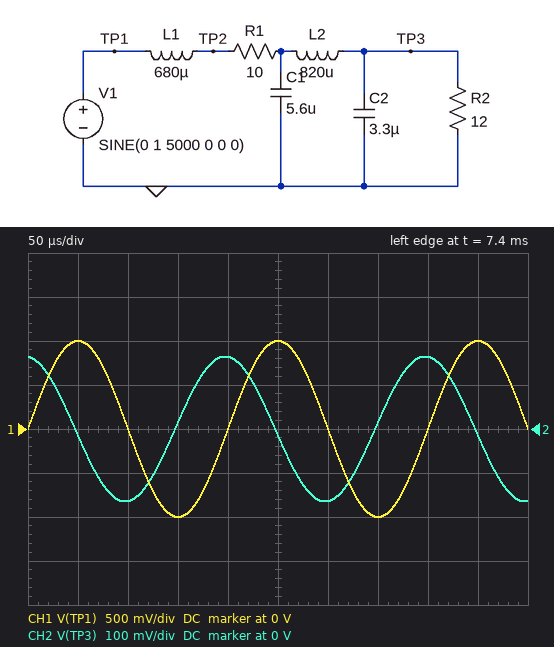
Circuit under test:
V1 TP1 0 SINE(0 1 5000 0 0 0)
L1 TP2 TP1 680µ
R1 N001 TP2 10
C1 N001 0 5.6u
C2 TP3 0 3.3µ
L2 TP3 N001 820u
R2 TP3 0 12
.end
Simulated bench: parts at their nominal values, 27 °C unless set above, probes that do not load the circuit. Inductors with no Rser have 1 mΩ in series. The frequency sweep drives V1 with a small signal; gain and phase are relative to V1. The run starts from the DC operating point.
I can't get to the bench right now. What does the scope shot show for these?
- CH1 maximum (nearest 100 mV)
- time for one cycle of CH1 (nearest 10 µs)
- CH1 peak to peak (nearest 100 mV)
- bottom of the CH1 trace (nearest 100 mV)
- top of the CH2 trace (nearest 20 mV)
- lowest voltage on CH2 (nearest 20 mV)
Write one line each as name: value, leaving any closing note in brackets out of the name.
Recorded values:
CH1 maximum: 1.0 V
time for one cycle of CH1: 200 µs
CH1 peak to peak: 2.0 V
bottom of the CH1 trace: -1.0 V
top of the CH2 trace: 160 mV
lowest voltage on CH2: -160 mV
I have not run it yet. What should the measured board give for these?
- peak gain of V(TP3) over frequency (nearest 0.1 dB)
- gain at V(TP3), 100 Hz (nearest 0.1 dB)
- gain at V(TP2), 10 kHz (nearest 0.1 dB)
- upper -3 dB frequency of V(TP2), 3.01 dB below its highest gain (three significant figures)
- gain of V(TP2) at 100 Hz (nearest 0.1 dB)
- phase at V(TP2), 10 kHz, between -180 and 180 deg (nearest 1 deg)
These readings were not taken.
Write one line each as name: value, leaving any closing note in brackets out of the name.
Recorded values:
peak gain of V(TP3) over frequency: -5.3 dB
gain at V(TP3), 100 Hz: -5.3 dB
gain at V(TP2), 10 kHz: -11.9 dB
upper -3 dB frequency of V(TP2), 3.01 dB below its highest gain: 4.70 kHz
gain of V(TP2) at 100 Hz: 0 dB
phase at V(TP2), 10 kHz, between -180 and 180 deg: -93 deg
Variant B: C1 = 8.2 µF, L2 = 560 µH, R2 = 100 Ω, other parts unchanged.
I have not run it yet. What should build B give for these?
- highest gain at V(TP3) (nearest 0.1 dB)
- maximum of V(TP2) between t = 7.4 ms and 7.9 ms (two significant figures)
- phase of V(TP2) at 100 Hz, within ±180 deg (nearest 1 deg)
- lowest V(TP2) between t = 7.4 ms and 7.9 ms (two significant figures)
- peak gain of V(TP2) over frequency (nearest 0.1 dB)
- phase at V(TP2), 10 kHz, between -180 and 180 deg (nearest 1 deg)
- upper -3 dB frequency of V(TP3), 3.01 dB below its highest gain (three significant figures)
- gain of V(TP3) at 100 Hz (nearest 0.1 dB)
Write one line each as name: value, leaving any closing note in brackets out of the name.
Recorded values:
highest gain at V(TP3): 3.5 dB
maximum of V(TP2) between t = 7.4 ms and 7.9 ms: 740 mV
phase of V(TP2) at 100 Hz, within ±180 deg: 0 deg
lowest V(TP2) between t = 7.4 ms and 7.9 ms: -740 mV
peak gain of V(TP2) over frequency: 1.9 dB
phase at V(TP2), 10 kHz, between -180 and 180 deg: -88 deg
upper -3 dB frequency of V(TP3), 3.01 dB below its highest gain: 4.70 kHz
gain of V(TP3) at 100 Hz: -0.8 dB
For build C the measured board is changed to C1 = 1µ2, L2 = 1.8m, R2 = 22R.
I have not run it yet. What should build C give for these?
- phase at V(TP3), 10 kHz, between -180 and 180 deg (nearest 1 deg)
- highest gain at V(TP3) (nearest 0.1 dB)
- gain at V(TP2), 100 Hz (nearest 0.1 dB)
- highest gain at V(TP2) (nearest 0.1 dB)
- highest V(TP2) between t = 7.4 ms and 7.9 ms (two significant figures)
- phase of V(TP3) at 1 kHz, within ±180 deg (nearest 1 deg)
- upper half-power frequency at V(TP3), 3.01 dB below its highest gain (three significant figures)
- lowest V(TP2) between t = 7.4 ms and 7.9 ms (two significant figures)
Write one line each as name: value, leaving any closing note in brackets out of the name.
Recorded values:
phase at V(TP3), 10 kHz, between -180 and 180 deg: 33 deg
highest gain at V(TP3): -3.1 dB
gain at V(TP2), 100 Hz: 0 dB
highest gain at V(TP2): 9.4 dB
highest V(TP2) between t = 7.4 ms and 7.9 ms: 1.5 V
phase of V(TP3) at 1 kHz, within ±180 deg: -42 deg
upper half-power frequency at V(TP3), 3.01 dB below its highest gain: 2.45 kHz
lowest V(TP2) between t = 7.4 ms and 7.9 ms: -1.5 V
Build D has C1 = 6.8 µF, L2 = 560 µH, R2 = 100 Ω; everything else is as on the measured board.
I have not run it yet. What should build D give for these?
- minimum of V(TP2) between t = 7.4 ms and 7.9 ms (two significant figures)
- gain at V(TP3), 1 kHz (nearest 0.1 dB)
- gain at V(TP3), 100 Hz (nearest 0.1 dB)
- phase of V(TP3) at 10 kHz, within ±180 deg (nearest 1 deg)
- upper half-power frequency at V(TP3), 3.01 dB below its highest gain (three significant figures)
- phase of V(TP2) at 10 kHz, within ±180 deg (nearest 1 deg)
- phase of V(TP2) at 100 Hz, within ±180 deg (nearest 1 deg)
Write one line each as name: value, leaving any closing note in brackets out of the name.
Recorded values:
minimum of V(TP2) between t = 7.4 ms and 7.9 ms: -1.0 V
gain at V(TP3), 1 kHz: -0.1 dB
gain at V(TP3), 100 Hz: -0.8 dB
phase of V(TP3) at 10 kHz, within ±180 deg: 17 deg
upper half-power frequency at V(TP3), 3.01 dB below its highest gain: 4.88 kHz
phase of V(TP2) at 10 kHz, within ±180 deg: -90 deg
phase of V(TP2) at 100 Hz, within ±180 deg: 0 deg
